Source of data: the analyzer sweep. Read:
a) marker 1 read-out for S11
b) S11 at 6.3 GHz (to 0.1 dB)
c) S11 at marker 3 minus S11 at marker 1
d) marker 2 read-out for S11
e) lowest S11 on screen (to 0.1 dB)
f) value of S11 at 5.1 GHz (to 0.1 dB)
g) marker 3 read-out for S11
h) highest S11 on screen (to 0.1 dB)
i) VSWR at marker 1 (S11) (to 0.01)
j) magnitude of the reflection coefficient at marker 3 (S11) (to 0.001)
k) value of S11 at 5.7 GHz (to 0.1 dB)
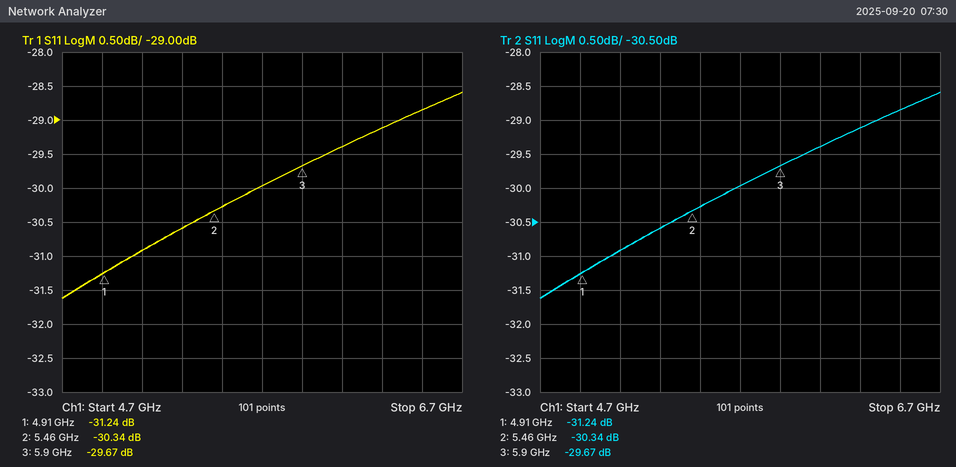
-31.24 dB
-29.1 dB
1.57 dB
-30.34 dB
-31.6 dB
-30.9 dB
-29.67 dB
-28.6 dB
1.06
0.033
-30.0 dB
